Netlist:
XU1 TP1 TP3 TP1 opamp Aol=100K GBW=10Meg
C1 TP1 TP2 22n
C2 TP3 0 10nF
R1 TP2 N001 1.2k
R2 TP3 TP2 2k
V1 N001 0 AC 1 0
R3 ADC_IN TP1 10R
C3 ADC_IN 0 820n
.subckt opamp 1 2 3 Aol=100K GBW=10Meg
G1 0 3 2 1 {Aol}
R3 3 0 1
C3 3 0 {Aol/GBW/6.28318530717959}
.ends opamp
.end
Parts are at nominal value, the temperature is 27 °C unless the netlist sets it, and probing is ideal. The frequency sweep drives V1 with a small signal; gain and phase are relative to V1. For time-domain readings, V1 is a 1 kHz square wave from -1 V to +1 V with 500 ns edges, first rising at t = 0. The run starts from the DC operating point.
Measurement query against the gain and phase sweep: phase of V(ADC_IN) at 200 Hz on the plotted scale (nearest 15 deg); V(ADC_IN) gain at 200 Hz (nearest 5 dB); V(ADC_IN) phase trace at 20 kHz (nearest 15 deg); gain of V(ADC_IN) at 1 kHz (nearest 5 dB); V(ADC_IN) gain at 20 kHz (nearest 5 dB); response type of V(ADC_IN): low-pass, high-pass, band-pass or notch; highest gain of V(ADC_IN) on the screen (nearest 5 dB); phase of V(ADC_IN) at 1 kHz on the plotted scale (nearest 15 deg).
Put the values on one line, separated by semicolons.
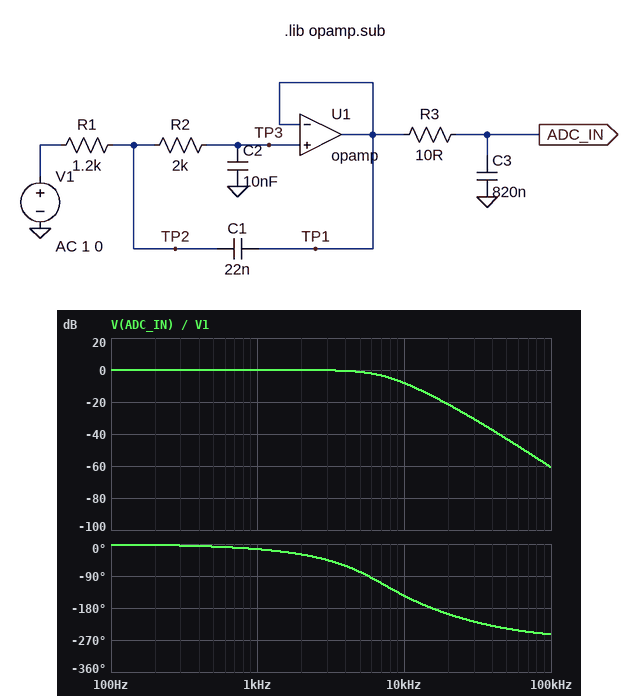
0 deg; 0 dB; -195 deg; 0 dB; -20 dB; low-pass; 0 dB; -15 deg
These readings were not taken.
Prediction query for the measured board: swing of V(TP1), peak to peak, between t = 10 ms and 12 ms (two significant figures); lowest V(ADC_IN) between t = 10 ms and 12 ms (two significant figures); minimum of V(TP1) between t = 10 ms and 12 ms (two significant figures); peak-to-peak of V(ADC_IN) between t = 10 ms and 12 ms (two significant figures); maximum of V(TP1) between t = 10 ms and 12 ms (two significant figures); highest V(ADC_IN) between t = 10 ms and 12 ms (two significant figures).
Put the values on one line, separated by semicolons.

2.2 V; -1.1 V; -1.1 V; 2.2 V; 1.1 V; 1.1 V
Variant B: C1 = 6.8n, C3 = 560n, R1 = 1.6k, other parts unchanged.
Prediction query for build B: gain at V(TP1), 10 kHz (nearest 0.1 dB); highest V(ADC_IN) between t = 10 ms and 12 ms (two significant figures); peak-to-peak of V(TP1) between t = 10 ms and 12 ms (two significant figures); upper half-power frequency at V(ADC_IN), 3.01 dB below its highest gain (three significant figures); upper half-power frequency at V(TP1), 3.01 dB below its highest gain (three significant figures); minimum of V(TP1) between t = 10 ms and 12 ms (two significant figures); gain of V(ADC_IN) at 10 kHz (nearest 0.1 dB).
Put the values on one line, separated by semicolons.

-7.1 dB; 1.0 V; 2.0 V; 5.11 kHz; 5.27 kHz; -1.0 V; -7.6 dB
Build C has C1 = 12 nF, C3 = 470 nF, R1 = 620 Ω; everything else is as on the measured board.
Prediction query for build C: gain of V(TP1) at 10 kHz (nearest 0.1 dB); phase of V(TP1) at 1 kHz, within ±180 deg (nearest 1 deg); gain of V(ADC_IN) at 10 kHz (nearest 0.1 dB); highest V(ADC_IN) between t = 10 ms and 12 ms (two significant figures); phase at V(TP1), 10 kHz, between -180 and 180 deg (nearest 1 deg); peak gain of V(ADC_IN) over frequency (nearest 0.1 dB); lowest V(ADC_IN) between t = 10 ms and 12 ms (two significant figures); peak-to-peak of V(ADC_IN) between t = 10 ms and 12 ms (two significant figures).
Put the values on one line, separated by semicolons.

-4.6 dB; -9 deg; -5.0 dB; 1.0 V; -76 deg; 0 dB; -1.0 V; 2.0 V
